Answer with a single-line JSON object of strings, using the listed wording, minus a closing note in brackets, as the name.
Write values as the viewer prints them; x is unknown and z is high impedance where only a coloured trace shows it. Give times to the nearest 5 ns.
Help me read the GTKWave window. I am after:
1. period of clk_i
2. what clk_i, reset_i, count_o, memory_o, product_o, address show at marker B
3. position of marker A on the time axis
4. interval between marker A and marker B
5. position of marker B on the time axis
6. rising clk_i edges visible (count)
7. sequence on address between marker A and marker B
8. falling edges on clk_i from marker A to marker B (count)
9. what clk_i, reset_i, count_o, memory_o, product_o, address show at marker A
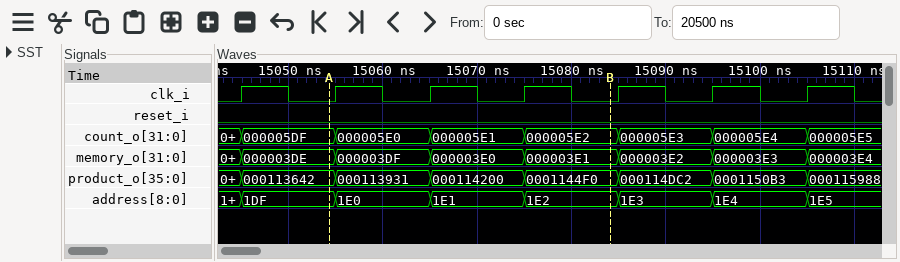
{"period of clk_i": "10 ns", "what clk_i, reset_i, count_o, memory_o, product_o, address show at marker B": "clk_i=0, reset_i=0, count_o=000005E2, memory_o=000003E1, product_o=0001144F0, address=1E2", "position of marker A on the time axis": "15055 ns", "interval between marker A and marker B": "30 ns", "position of marker B on the time axis": "15085 ns", "rising clk_i edges visible": "7", "sequence on address between marker A and marker B": "1DF, 1E0, 1E1, 1E2", "falling edges on clk_i from marker A to marker B": "3", "what clk_i, reset_i, count_o, memory_o, product_o, address show at marker A": "clk_i=0, reset_i=0, count_o=000005DF, memory_o=000003DE, product_o=000113642, address=1DF"}
